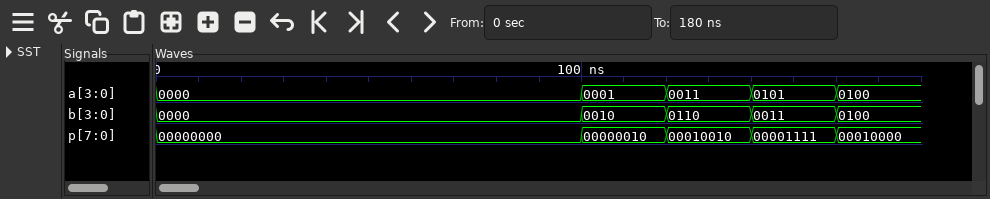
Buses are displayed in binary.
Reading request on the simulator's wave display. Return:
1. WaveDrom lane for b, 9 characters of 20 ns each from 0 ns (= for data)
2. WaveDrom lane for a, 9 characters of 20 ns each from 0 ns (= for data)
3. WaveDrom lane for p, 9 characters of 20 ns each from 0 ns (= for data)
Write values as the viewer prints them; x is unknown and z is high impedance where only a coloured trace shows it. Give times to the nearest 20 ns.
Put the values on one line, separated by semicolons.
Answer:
{name: 'b', wave: '=....====', data: '0000 0010 0110 0011 0100'}; {name: 'a', wave: '=....====', data: '0000 0001 0011 0101 0100'}; {name: 'p', wave: '=....====', data: '00000000 00000010 00010010 00001111 00010000'}
